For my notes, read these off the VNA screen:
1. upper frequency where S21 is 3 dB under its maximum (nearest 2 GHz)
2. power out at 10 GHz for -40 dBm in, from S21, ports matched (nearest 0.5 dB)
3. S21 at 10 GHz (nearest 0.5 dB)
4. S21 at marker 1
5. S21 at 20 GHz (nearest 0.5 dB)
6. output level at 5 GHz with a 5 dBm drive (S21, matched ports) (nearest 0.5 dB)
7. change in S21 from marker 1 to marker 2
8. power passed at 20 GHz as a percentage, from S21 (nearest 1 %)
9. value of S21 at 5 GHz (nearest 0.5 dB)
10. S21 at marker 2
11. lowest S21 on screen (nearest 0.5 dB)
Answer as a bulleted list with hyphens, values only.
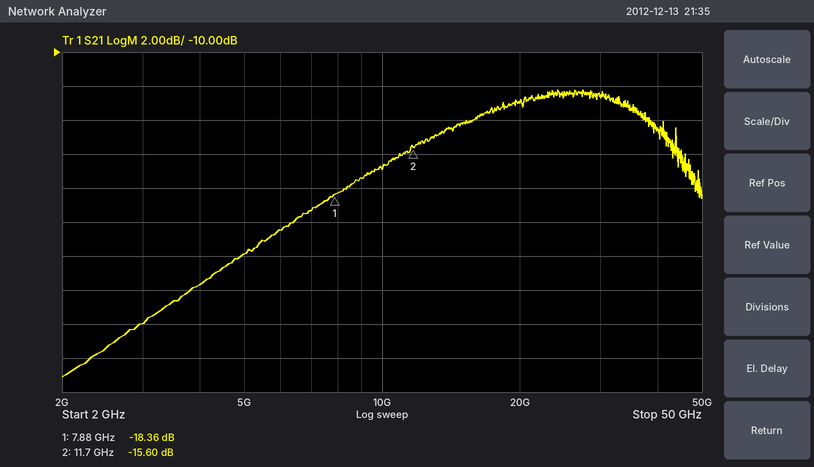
- 42 GHz
- -57.0 dBm
- -17.0 dB
- -18.36 dB
- -13.0 dB
- -17.0 dBm
- 2.76 dB
- 5 %
- -22.0 dB
- -15.60 dB
- -29.0 dB
